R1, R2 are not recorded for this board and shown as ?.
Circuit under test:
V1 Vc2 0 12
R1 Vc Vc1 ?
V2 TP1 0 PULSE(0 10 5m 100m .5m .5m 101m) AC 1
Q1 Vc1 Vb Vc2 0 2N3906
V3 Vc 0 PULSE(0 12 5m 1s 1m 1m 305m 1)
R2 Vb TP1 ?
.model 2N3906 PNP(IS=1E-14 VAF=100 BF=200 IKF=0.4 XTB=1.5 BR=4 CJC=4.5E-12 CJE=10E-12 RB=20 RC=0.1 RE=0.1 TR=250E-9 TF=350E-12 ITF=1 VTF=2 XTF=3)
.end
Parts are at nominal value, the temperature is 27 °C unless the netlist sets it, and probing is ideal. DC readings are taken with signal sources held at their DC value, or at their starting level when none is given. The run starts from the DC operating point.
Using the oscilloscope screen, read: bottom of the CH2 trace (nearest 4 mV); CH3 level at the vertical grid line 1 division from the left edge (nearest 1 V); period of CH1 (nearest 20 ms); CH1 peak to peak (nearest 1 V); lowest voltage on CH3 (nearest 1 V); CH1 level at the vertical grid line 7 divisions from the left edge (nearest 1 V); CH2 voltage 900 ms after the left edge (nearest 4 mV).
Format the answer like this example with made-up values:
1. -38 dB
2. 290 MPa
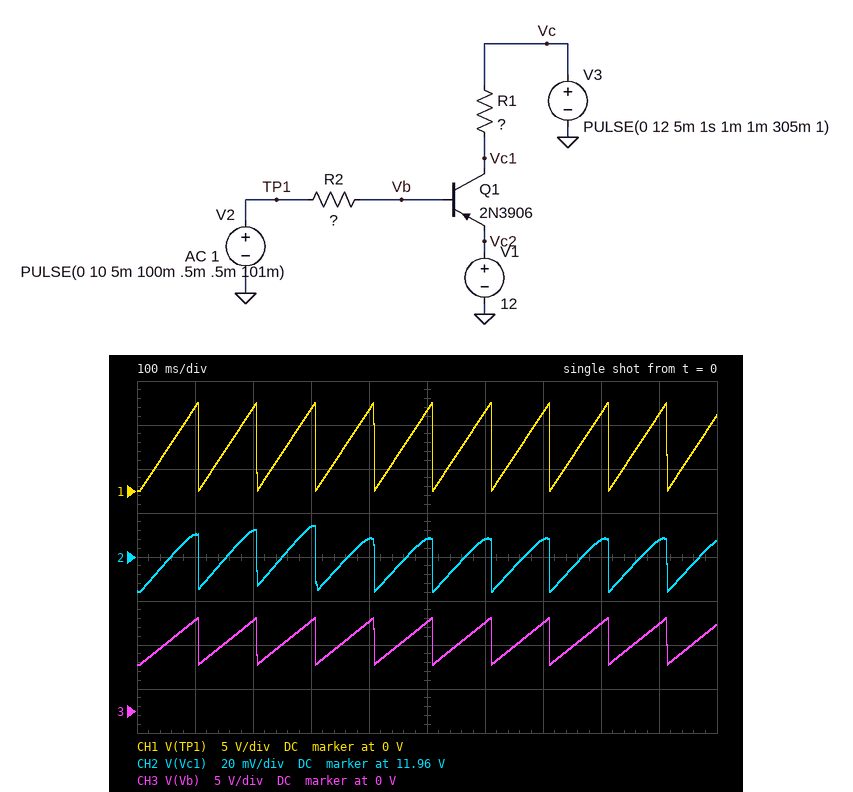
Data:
1. 11.944 V
2. 10 V
3. 100 ms
4. 10 V
5. 5 V
6. 9 V
7. 11.968 V
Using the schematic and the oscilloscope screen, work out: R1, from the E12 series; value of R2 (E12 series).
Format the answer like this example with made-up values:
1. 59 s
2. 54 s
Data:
1. 220 Ω
2. 18 Ω
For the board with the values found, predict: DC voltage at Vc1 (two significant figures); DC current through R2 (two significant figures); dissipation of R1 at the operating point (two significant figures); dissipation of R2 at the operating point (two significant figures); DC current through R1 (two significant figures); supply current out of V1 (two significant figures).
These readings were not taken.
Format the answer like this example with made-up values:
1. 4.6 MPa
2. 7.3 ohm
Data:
1. 12 V
2. 290 mA
3. 650 mW
4. 1.5 W
5. 54 mA
6. 350 mA
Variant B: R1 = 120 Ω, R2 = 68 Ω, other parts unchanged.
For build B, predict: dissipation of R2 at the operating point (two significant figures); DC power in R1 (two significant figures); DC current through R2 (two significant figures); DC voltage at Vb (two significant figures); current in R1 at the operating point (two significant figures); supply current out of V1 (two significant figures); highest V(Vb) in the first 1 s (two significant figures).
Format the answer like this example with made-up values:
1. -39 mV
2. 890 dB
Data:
1. 1.1 W
2. 1.2 W
3. 130 mA
4. 8.6 V
5. 100 mA
6. 230 mA
7. 11 V
